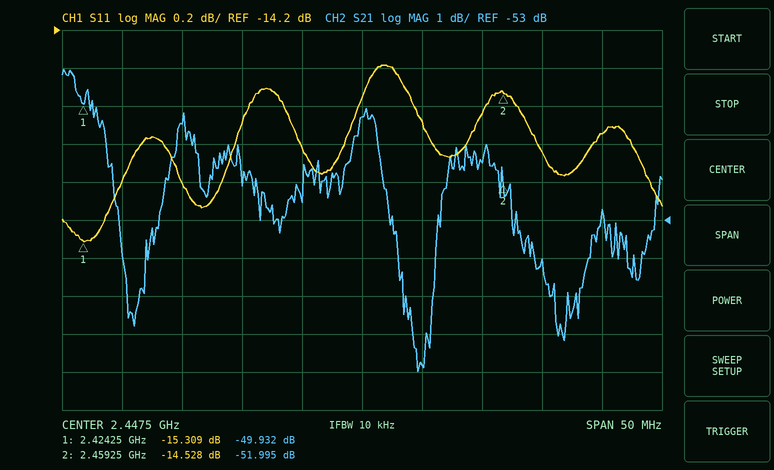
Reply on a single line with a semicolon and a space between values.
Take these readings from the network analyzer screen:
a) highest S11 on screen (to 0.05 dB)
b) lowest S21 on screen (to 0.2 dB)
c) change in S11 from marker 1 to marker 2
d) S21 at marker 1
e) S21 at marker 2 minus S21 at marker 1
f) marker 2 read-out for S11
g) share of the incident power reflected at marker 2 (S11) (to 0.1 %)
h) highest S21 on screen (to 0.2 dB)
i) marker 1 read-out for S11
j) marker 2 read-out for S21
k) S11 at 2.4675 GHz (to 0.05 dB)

-14.40 dB; -57.0 dB; 0.781 dB; -49.932 dB; -2.063 dB; -14.528 dB; 3.5 %; -49.0 dB; -15.309 dB; -51.995 dB; -14.75 dB
